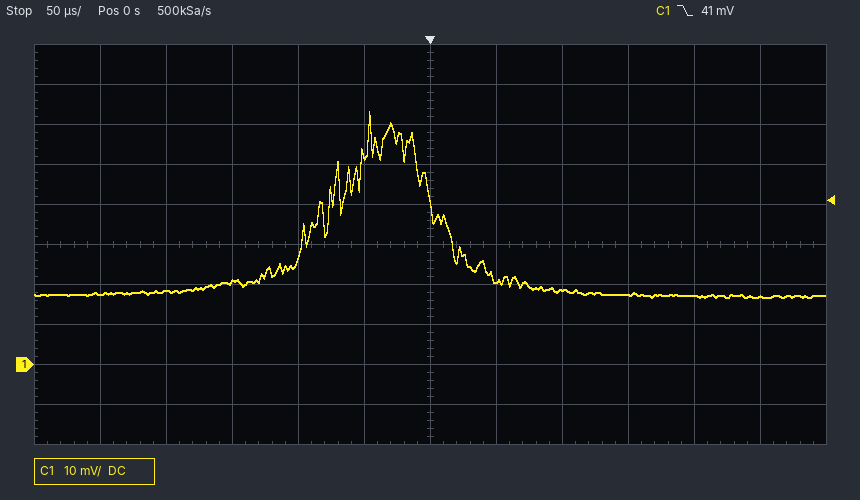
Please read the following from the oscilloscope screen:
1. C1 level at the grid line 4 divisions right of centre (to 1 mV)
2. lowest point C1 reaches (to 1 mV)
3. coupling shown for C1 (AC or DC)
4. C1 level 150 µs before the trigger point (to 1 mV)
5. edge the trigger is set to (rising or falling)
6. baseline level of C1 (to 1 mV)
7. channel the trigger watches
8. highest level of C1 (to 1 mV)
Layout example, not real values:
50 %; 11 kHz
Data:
17 mV; 17 mV; DC; 21 mV; falling; 18 mV; C1; 63 mV
